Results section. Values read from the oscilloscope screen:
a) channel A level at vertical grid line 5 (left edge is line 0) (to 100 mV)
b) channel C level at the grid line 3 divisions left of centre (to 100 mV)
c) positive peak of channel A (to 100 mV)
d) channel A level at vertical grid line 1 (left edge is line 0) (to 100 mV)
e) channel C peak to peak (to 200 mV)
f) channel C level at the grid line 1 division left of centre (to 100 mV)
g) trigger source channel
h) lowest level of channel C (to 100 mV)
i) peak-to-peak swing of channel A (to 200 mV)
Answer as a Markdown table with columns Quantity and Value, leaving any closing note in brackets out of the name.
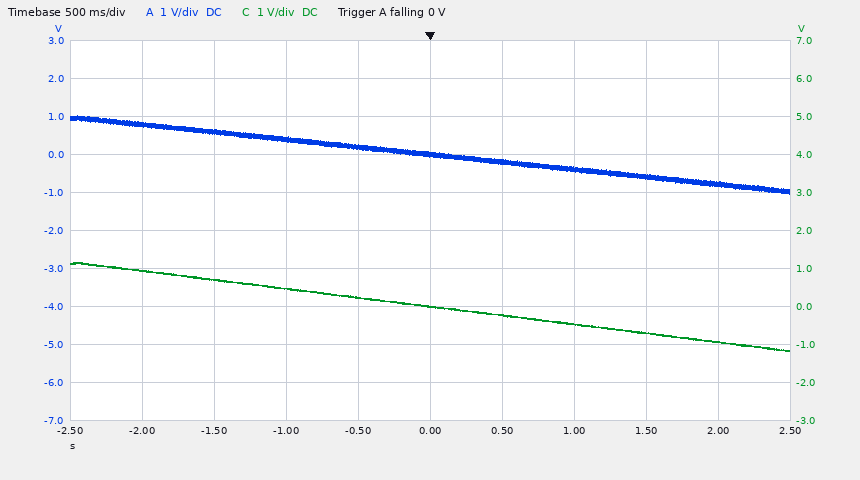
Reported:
| Quantity | Value |
|---|---|
| channel A level at vertical grid line 5 (left edge is line 0) | 0.0 V |
| channel C level at the grid line 3 divisions left of centre | 700 mV |
| positive peak of channel A | 1.0 V |
| channel A level at vertical grid line 1 (left edge is line 0) | 800 mV |
| channel C peak to peak | 2.4 V |
| channel C level at the grid line 1 division left of centre | 200 mV |
| trigger source channel | channel A |
| lowest level of channel C | -1.2 V |
| peak-to-peak swing of channel A | 2.0 V |
